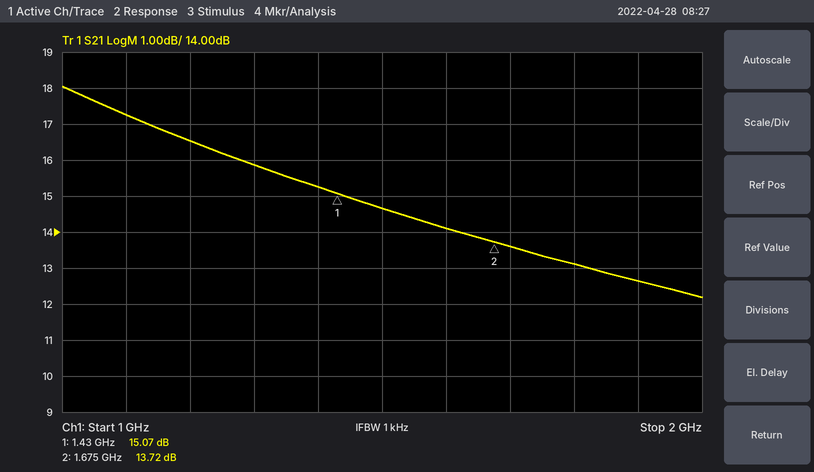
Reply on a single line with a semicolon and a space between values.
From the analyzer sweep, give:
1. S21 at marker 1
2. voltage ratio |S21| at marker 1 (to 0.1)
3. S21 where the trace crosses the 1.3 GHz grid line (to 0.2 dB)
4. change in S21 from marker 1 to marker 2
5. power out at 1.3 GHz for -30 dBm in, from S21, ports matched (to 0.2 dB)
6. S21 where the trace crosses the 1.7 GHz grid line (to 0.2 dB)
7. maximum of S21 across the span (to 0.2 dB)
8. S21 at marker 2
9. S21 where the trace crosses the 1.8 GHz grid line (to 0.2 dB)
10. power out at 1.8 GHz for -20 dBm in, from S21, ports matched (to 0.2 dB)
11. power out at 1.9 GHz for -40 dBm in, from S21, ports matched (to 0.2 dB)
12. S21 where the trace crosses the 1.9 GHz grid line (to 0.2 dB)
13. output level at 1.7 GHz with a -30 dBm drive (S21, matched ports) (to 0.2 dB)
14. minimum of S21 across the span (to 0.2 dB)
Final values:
15.07 dB; 5.7; 15.8 dB; -1.35 dB; -14.2 dBm; 13.6 dB; 18.0 dB; 13.72 dB; 13.2 dB; -6.8 dBm; -27.4 dBm; 12.6 dB; -16.4 dBm; 12.2 dB
